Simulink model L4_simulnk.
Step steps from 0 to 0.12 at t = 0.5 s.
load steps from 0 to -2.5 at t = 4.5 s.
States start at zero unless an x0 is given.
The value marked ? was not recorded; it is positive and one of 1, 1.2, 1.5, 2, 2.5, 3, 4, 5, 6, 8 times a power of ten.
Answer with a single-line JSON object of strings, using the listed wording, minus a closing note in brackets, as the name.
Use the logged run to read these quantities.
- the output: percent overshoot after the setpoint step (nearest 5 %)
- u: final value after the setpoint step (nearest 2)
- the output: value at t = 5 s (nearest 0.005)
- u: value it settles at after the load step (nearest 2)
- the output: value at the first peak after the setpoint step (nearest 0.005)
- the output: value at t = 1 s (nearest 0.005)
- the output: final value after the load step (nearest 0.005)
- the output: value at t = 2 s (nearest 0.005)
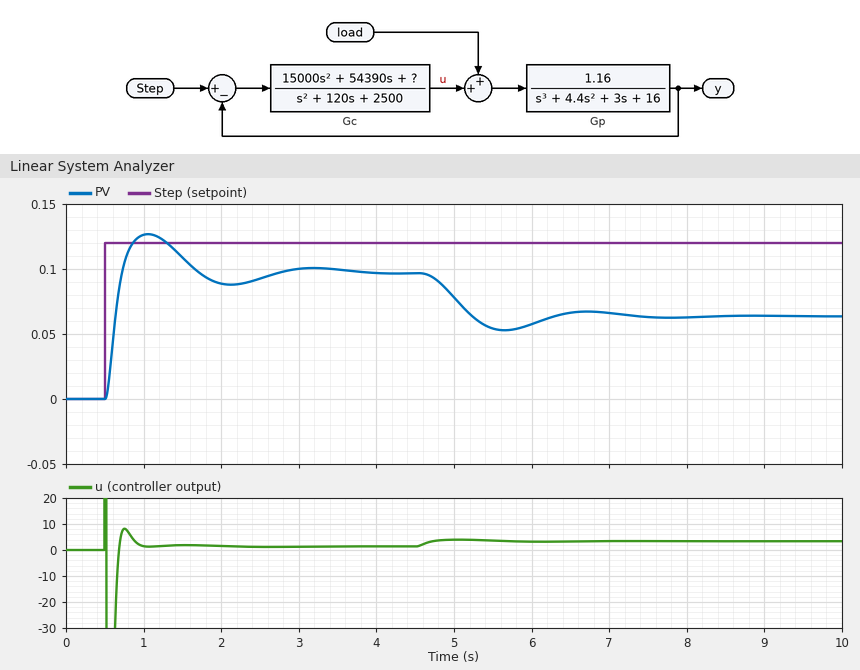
{"the output: percent overshoot after the setpoint step": "30 %", "u: final value after the setpoint step": "2", "the output: value at t = 5 s": "0.080", "u: value it settles at after the load step": "4", "the output: value at the first peak after the setpoint step": "0.125", "the output: value at t = 1 s": "0.125", "the output: final value after the load step": "0.065", "the output: value at t = 2 s": "0.090"}
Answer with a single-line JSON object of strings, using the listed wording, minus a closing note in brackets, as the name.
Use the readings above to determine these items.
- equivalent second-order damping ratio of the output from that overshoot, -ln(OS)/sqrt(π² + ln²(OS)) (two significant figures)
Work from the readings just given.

{"equivalent second-order damping ratio of the output from that overshoot, -ln(OS)/sqrt(π² + ln²(OS))": "0.36"}
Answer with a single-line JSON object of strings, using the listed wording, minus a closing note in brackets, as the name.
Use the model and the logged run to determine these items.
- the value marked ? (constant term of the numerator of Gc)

{"the value marked ?": "150000"}
